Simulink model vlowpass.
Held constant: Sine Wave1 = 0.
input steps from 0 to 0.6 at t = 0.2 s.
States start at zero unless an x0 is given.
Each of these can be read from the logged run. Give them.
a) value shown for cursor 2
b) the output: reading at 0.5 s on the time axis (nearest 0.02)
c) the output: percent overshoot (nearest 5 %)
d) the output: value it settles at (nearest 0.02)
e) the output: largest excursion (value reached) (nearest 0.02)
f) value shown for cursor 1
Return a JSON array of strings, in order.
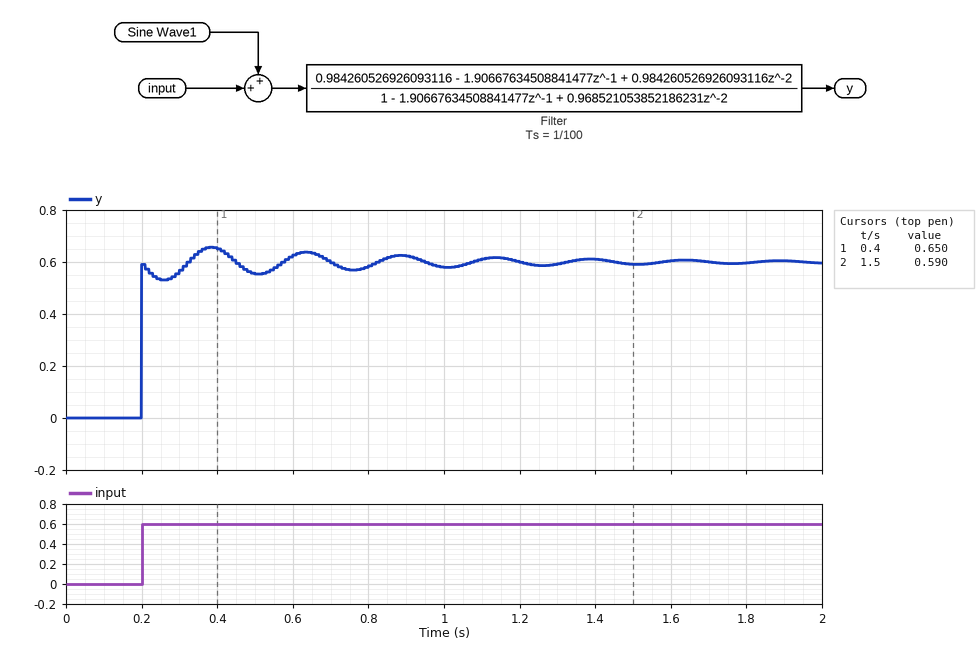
["0.590", "0.56", "10 %", "0.60", "0.66", "0.650"]
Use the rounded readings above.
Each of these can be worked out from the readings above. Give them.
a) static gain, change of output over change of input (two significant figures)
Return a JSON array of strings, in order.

["1.0"]
